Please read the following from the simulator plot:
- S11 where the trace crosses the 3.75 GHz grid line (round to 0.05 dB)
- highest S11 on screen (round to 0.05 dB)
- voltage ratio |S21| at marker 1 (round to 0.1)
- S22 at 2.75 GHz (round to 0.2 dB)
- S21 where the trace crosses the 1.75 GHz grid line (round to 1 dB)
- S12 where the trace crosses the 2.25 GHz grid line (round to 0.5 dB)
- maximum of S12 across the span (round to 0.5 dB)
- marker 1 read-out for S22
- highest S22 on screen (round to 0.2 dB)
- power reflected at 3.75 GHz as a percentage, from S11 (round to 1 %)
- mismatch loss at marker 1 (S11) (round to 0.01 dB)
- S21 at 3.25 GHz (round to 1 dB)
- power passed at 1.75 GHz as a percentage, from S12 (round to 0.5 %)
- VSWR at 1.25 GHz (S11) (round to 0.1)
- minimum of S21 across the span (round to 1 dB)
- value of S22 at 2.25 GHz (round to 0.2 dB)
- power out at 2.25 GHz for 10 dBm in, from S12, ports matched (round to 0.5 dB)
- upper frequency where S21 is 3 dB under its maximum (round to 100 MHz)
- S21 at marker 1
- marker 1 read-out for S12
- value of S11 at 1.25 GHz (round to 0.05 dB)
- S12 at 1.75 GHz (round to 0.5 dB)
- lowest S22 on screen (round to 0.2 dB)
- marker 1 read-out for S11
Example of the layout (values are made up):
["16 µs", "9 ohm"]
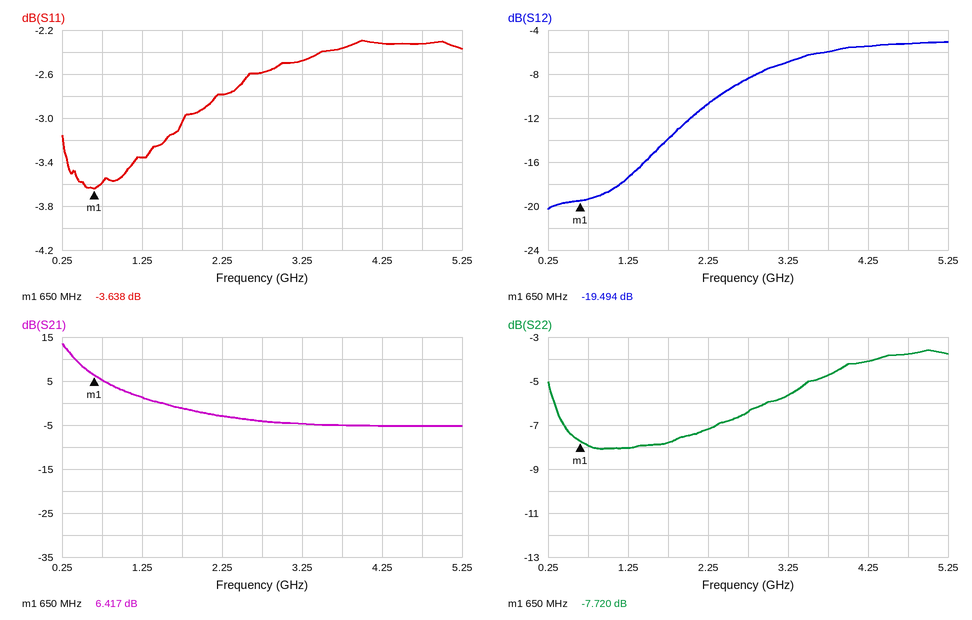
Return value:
["-2.35 dB", "-2.30 dB", "2.1", "-6.4 dB", "-1 dB", "-10.5 dB", "-5.0 dB", "-7.720 dB", "-3.6 dB", "58 %", "2.46 dB", "-5 dB", "4.0 %", "5.2", "-5 dB", "-7.2 dB", "-0.5 dBm", "400 MHz", "6.417 dB", "-19.494 dB", "-3.35 dB", "-14.0 dB", "-8.0 dB", "-3.638 dB"]
